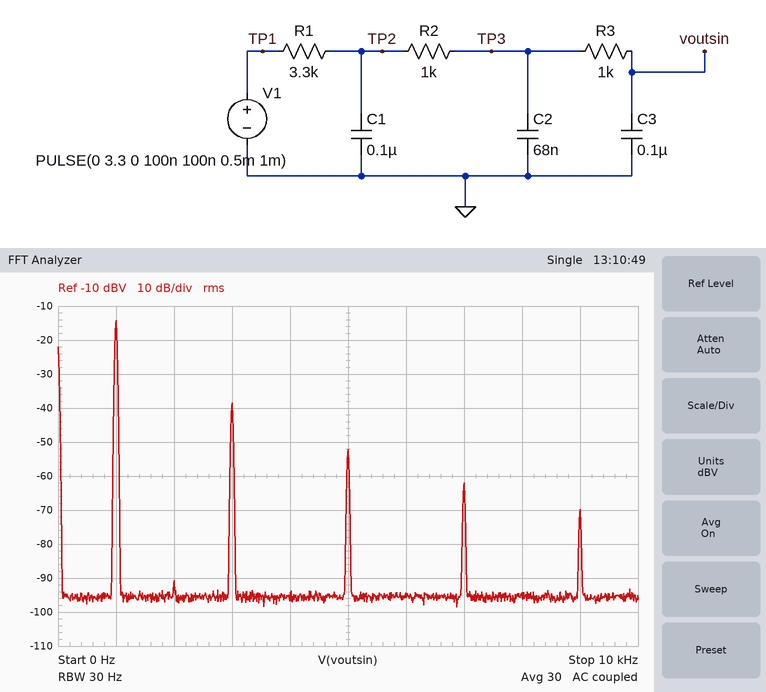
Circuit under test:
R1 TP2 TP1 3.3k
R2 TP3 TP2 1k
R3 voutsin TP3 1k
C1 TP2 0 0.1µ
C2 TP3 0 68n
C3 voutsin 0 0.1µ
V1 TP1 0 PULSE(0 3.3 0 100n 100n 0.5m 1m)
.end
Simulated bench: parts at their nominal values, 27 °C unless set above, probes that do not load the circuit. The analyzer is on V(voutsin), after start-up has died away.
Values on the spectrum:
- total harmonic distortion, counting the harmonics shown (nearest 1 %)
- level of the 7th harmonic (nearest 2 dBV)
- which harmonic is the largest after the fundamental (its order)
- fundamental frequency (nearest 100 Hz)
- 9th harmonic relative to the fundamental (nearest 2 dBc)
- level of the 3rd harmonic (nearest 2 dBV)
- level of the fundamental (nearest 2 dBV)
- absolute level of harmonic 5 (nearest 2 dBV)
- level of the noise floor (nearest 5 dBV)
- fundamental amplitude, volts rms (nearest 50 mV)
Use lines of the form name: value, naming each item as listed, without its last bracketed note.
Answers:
total harmonic distortion, counting the harmonics shown: 6 %
level of the 7th harmonic: -62 dBV
which harmonic is the largest after the fundamental: 3
fundamental frequency: 1.0 kHz
9th harmonic relative to the fundamental: -56 dBc
level of the 3rd harmonic: -38 dBV
level of the fundamental: -14 dBV
absolute level of harmonic 5: -52 dBV
level of the noise floor: -95 dBV
fundamental amplitude, volts rms: 200 mV
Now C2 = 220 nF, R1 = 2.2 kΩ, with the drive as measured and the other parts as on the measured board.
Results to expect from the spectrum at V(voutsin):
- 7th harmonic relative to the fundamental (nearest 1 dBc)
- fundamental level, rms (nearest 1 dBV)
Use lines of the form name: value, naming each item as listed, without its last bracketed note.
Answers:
7th harmonic relative to the fundamental: -51 dBc
fundamental level, rms: -16 dBV
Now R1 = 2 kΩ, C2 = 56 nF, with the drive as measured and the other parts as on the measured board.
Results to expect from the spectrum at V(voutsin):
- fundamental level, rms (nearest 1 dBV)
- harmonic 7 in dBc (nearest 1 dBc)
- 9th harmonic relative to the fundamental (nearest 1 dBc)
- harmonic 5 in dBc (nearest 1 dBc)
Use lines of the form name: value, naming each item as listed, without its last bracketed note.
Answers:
fundamental level, rms: -10 dBV
harmonic 7 in dBc: -46 dBc
9th harmonic relative to the fundamental: -54 dBc
harmonic 5 in dBc: -37 dBc
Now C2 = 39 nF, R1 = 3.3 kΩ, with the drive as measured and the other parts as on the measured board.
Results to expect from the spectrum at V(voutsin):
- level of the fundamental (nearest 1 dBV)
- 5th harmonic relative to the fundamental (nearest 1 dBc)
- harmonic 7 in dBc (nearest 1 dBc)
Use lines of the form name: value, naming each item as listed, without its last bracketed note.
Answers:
level of the fundamental: -13 dBV
5th harmonic relative to the fundamental: -37 dBc
harmonic 7 in dBc: -46 dBc
